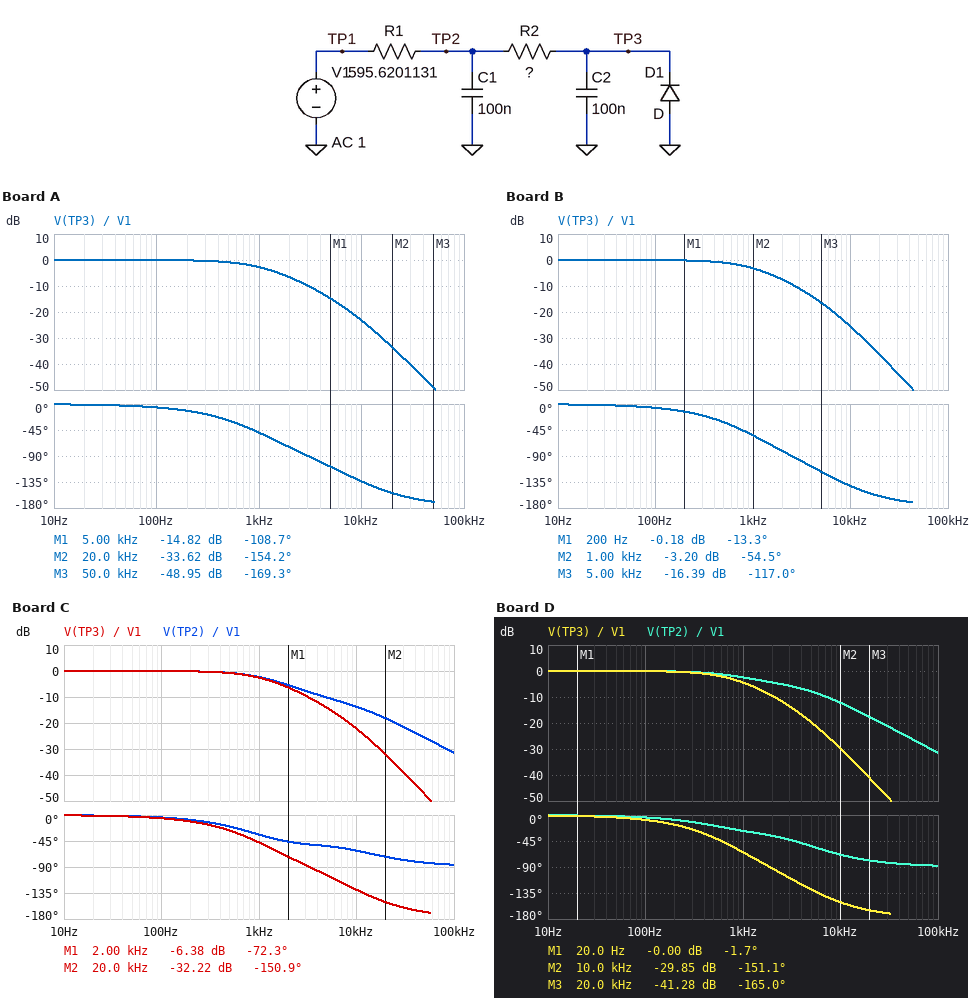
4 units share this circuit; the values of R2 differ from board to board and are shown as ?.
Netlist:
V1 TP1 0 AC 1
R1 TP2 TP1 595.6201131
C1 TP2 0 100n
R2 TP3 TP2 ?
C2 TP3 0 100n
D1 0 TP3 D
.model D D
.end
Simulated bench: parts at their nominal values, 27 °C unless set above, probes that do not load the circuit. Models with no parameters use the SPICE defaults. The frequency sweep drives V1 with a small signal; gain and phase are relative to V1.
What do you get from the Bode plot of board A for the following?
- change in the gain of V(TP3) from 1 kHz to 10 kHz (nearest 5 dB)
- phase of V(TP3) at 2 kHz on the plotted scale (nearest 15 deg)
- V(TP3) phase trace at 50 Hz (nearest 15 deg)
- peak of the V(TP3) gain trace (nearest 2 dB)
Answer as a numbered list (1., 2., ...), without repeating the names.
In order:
1. -20 dB
2. -75 deg
3. 0 deg
4. 0 dB
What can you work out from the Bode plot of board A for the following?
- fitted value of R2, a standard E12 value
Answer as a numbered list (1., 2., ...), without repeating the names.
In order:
1. 470 Ω
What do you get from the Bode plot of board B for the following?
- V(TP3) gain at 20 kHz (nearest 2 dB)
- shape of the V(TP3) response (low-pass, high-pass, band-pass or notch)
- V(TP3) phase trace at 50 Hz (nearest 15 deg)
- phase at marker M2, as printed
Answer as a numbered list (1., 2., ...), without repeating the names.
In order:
1. -36 dB
2. low-pass
3. 0 deg
4. -54.5 deg
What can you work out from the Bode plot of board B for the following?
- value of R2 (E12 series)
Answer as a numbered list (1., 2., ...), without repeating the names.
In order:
1. 680 Ω
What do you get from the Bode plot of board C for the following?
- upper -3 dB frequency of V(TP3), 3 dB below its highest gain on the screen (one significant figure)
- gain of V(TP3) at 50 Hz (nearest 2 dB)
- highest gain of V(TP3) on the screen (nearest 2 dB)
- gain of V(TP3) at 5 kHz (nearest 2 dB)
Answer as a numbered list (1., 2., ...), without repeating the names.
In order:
1. 1 kHz
2. 0 dB
3. 0 dB
4. -14 dB
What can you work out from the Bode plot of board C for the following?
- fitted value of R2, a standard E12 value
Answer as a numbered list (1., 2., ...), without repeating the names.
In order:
1. 390 Ω
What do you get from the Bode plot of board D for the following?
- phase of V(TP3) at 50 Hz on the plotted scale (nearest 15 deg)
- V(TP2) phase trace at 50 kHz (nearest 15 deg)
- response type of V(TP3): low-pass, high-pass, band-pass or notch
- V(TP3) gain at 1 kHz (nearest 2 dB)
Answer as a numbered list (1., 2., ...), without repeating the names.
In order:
1. 0 deg
2. -90 deg
3. low-pass
4. -4 dB
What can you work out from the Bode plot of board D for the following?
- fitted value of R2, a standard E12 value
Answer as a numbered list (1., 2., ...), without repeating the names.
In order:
1. 1.2 kΩ
